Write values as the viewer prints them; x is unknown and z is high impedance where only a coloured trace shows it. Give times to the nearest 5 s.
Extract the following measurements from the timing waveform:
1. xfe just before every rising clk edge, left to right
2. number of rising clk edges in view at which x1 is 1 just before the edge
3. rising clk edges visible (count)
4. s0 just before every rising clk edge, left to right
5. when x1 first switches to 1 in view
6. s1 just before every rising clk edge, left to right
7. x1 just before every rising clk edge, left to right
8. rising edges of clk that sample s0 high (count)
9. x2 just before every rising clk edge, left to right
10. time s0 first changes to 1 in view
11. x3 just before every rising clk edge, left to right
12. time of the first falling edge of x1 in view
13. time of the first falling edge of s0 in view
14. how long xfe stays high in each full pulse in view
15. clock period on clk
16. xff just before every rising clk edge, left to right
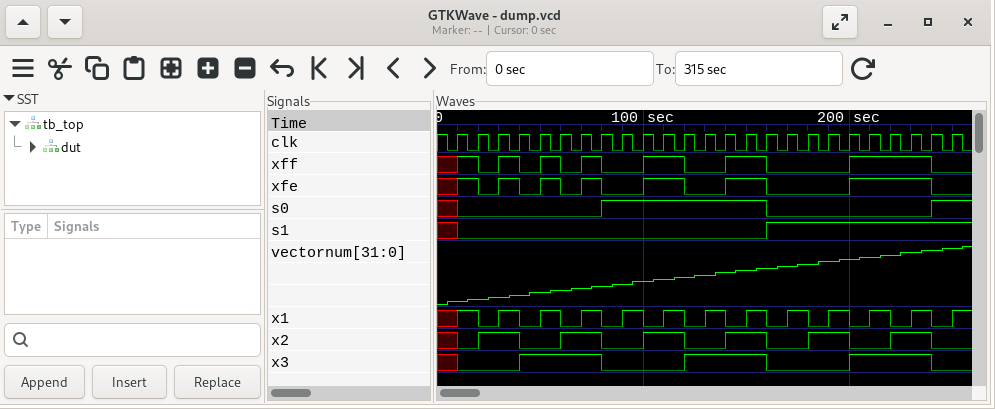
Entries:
x 1 0 1 0 1 0 1 0 0 1 1 0 0 1 1 0 0 0 0 1 1 1 1 0
12
25
x 0 0 0 0 0 0 0 1 1 1 1 1 1 1 1 0 0 0 0 0 0 0 0 1
10 s
x 0 0 0 0 0 0 0 0 0 0 0 0 0 0 0 1 1 1 1 1 1 1 1 1
x 1 0 1 0 1 0 1 0 1 0 1 0 1 0 1 0 1 0 1 0 1 0 1 0
9
x 0 1 1 0 0 1 1 0 0 1 1 0 0 1 1 0 0 1 1 0 0 1 1 0
80 s
x 0 0 0 1 1 1 1 0 0 0 0 1 1 1 1 0 0 0 0 1 1 1 1 0
20 s
160 s
10 s, 10 s, 10 s, 20 s, 20 s, 40 s
10 s
x 1 0 1 0 1 0 1 0 0 1 1 0 0 1 1 0 0 0 0 1 1 1 1 0
